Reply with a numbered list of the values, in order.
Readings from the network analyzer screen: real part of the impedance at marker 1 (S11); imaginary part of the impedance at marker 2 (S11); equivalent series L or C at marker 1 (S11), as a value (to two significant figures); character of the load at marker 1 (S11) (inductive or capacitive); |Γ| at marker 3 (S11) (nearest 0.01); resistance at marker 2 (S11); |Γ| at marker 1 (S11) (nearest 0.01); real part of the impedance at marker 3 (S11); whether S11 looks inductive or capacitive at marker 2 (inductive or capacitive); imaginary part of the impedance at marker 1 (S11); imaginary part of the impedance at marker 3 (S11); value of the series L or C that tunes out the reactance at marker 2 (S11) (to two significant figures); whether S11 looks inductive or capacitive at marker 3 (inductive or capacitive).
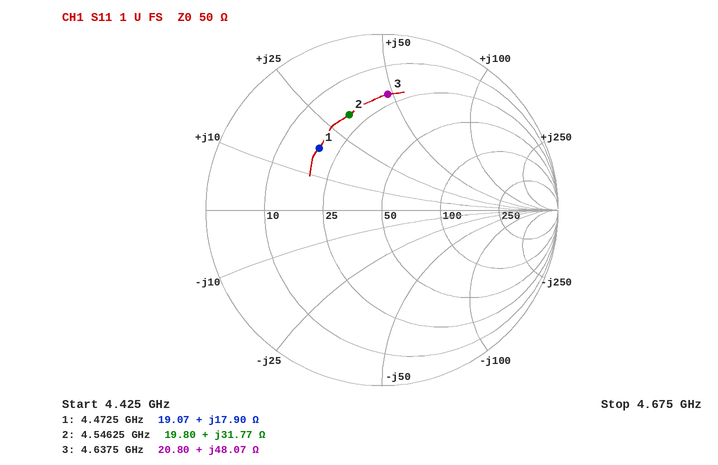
1. 19.07 Ω
2. +31.77 Ω
3. 640 pH
4. inductive
5. 0.66
6. 19.80 Ω
7. 0.50
8. 20.80 Ω
9. inductive
10. +17.90 Ω
11. +48.07 Ω
12. 1.1 pF
13. inductive
